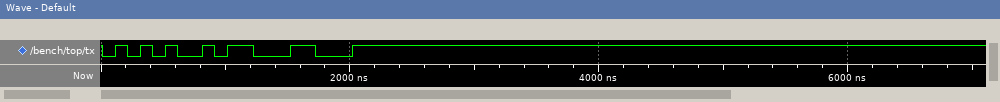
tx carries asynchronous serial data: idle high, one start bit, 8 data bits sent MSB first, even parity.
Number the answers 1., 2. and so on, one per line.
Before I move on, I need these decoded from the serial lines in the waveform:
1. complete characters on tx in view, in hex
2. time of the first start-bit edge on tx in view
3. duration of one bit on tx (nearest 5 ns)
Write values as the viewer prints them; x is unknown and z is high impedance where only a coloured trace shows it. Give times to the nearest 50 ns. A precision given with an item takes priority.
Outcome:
1. A9, 31
2. 0 ns
3. 100 ns
